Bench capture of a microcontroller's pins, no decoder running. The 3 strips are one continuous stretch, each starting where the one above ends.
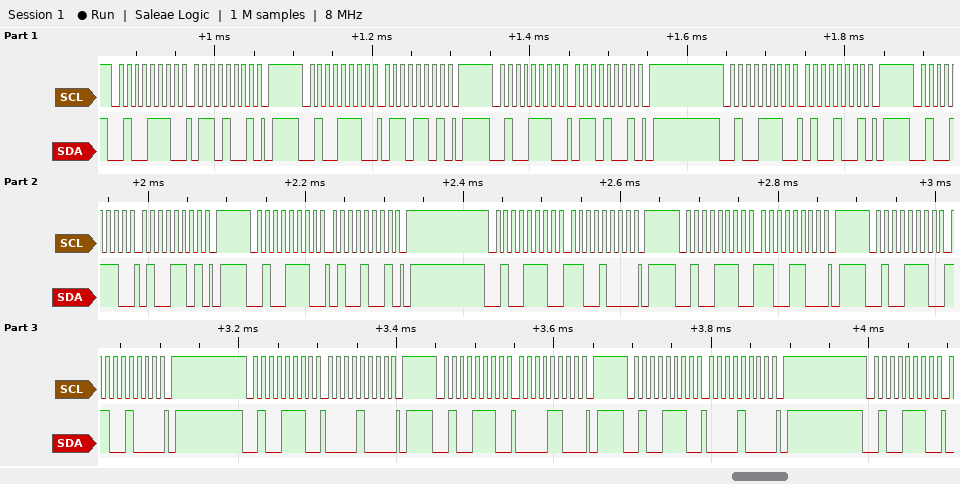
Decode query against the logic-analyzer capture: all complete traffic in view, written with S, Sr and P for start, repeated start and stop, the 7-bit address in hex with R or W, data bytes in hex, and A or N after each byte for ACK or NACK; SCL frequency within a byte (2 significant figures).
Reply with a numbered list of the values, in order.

1. S 27W A 69 A P S 27W A 6D A P S 27W A 69 A P S 27W A 49 A P S 27W A 4D A P S 27W A 49 A P S 27W A C8 A P S 27W A CC A P S 27W A C8 A P S 27W A 08 A P S 27W A 0C A P S 27W A 08 A P S 27W A
2. 100 kHz
